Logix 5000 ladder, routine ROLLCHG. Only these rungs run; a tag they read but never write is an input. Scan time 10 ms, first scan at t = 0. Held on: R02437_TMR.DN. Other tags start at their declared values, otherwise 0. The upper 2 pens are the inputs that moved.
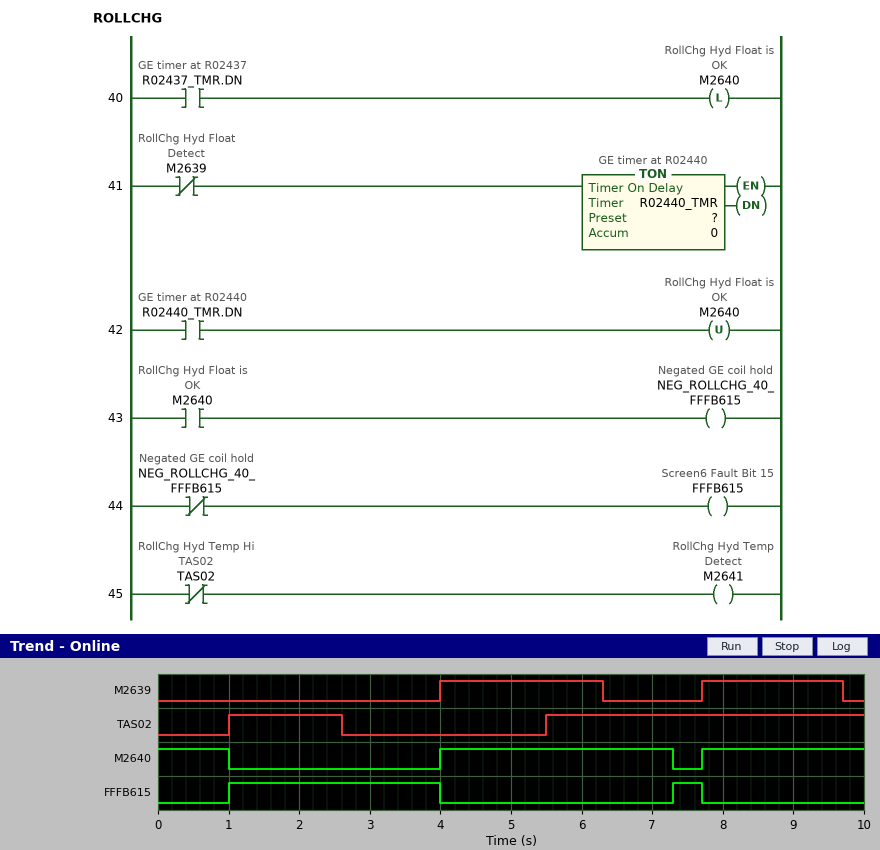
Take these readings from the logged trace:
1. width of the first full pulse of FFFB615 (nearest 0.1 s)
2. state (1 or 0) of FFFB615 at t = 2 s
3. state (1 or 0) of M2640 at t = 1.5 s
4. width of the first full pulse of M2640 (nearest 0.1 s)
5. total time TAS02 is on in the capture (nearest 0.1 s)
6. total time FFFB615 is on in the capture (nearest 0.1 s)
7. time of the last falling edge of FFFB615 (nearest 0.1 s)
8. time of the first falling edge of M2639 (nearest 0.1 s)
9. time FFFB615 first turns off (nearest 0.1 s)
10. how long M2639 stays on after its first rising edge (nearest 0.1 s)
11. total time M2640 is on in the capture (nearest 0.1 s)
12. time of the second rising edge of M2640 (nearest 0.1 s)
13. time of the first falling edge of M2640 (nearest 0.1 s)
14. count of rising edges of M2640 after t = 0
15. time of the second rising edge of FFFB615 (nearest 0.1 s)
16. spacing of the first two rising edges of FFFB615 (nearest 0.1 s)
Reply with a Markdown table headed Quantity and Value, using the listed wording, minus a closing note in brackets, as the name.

| Quantity | Value |
|---|---|
| width of the first full pulse of FFFB615 | 3.0 s |
| state (1 or 0) of FFFB615 at t = 2 s | 1 |
| state (1 or 0) of M2640 at t = 1.5 s | 0 |
| width of the first full pulse of M2640 | 3.3 s |
| total time TAS02 is on in the capture | 6.1 s |
| total time FFFB615 is on in the capture | 3.4 s |
| time of the last falling edge of FFFB615 | 7.7 s |
| time of the first falling edge of M2639 | 6.3 s |
| time FFFB615 first turns off | 4.0 s |
| how long M2639 stays on after its first rising edge | 2.3 s |
| total time M2640 is on in the capture | 6.6 s |
| time of the second rising edge of M2640 | 7.7 s |
| time of the first falling edge of M2640 | 1.0 s |
| count of rising edges of M2640 after t = 0 | 2 |
| time of the second rising edge of FFFB615 | 7.3 s |
| spacing of the first two rising edges of FFFB615 | 6.3 s |
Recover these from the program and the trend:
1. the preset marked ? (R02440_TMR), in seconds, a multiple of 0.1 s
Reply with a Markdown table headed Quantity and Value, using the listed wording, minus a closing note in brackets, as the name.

| Quantity | Value |
|---|---|
| the preset marked ? (R02440_TMR), in seconds, a multiple of 0.1 s | 1.0 s |
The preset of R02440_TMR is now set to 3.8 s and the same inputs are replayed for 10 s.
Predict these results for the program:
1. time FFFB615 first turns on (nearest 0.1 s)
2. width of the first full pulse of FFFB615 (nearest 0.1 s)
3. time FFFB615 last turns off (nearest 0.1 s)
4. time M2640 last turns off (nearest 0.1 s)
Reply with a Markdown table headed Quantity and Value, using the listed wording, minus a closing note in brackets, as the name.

| Quantity | Value |
|---|---|
| time FFFB615 first turns on | 3.8 s |
| width of the first full pulse of FFFB615 | 0.2 s |
| time FFFB615 last turns off | 4.0 s |
| time M2640 last turns off | 3.8 s |
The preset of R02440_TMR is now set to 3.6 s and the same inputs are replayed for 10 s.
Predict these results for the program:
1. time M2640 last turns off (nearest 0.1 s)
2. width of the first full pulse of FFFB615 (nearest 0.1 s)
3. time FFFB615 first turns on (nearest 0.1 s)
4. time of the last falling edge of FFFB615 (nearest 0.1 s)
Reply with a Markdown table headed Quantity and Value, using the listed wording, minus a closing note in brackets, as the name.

| Quantity | Value |
|---|---|
| time M2640 last turns off | 3.6 s |
| width of the first full pulse of FFFB615 | 0.4 s |
| time FFFB615 first turns on | 3.6 s |
| time of the last falling edge of FFFB615 | 4.0 s |
